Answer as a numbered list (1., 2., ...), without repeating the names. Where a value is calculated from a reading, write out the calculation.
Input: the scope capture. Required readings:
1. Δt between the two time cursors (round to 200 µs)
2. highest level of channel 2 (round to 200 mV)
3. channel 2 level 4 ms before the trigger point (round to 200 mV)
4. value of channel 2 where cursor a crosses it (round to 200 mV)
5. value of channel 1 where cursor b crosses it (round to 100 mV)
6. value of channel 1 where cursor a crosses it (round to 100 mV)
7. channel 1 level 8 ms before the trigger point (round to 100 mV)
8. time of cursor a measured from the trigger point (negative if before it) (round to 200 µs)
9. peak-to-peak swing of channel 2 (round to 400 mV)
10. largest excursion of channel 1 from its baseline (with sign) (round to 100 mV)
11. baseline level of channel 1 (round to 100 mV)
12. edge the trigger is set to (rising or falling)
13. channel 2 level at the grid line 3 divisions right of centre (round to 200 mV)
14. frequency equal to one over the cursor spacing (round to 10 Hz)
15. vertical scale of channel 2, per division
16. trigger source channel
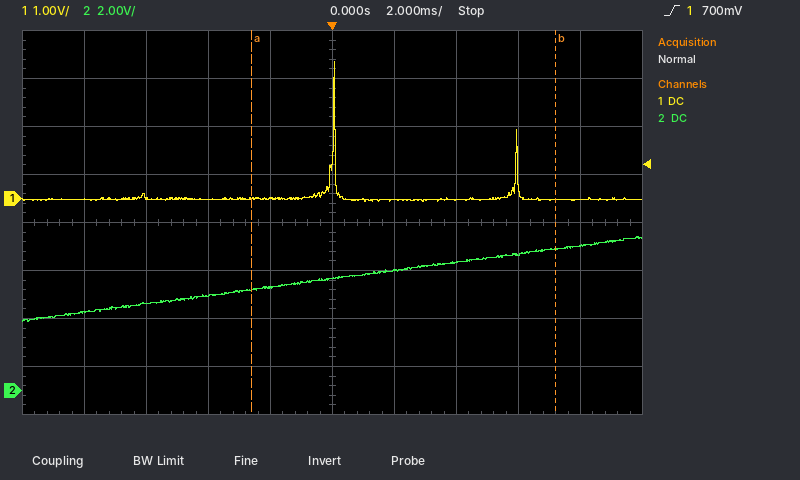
1. 9.8 ms
2. 6.4 V
3. 4.0 V
4. 4.2 V
5. 0.0 V
6. 0.0 V
7. 0.0 V
8. -2.6 ms
9. 3.6 V
10. +2.9 V
11. 0.0 V
12. rising
13. 5.6 V
14. 1 / 9.8 ms ≈ 100 Hz
15. 2 V
16. channel 1
